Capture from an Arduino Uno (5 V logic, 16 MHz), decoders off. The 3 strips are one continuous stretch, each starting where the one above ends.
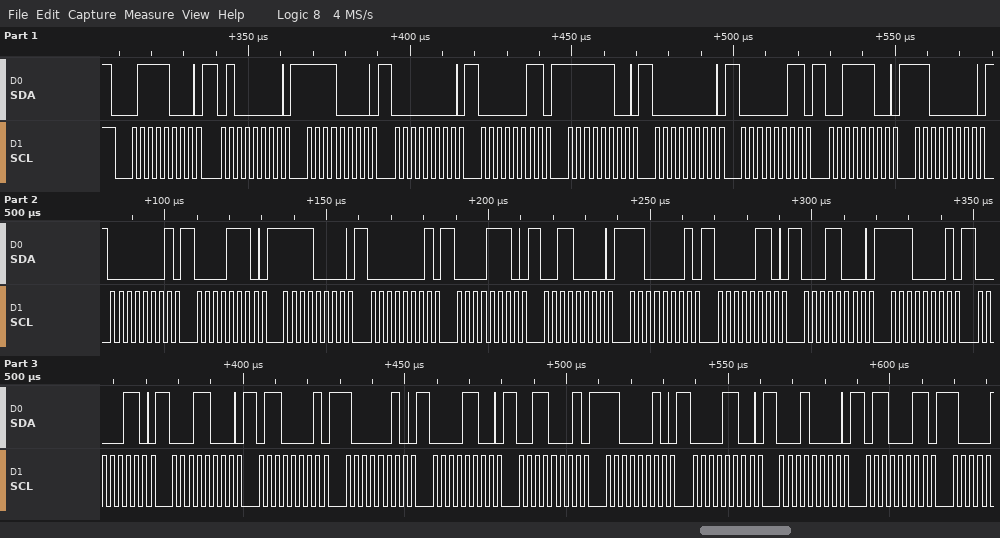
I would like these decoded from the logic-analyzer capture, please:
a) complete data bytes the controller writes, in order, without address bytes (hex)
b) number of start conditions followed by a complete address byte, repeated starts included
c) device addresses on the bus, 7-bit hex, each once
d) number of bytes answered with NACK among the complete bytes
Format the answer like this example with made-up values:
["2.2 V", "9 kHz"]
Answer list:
["40 F0 00 03 FC 00 03 3C C0 01 0E F0 01 0E 30 C1 06 18 E1 06 18 61 82 0C 31 C2 0C 10 63", "1", "0x3C", "0"]
